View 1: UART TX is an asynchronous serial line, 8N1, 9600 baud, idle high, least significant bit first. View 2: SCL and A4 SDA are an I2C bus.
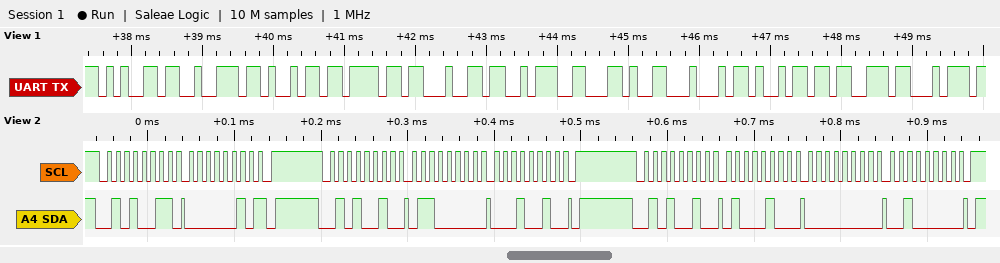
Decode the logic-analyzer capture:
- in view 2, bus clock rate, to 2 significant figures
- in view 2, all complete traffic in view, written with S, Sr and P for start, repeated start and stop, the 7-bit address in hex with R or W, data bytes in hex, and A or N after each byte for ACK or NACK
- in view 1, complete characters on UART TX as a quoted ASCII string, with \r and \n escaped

100 kHz
S 29R A 02 N P S 29W A 60 A 12 A P S 29W A 44 A 00 A 20 A P
"eriod:,Dist"
